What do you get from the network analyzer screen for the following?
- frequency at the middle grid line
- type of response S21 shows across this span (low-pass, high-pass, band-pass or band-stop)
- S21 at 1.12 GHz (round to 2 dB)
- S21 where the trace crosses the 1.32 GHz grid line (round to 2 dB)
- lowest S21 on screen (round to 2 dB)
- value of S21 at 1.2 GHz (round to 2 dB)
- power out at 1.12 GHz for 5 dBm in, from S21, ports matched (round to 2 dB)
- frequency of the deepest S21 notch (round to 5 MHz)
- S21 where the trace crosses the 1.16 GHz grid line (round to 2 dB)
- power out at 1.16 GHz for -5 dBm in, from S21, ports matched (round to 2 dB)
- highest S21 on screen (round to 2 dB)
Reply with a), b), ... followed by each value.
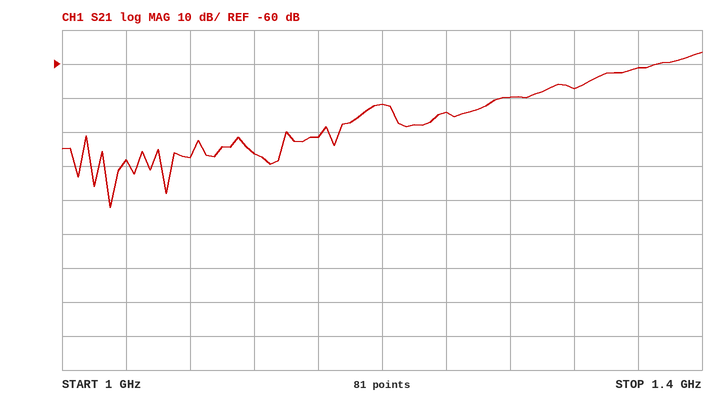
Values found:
a) 1.2 GHz
b) high-pass
c) -86 dB
d) -68 dB
e) -102 dB
f) -72 dB
g) -82 dBm
h) 1.030 GHz
i) -82 dB
j) -86 dBm
k) -56 dB
